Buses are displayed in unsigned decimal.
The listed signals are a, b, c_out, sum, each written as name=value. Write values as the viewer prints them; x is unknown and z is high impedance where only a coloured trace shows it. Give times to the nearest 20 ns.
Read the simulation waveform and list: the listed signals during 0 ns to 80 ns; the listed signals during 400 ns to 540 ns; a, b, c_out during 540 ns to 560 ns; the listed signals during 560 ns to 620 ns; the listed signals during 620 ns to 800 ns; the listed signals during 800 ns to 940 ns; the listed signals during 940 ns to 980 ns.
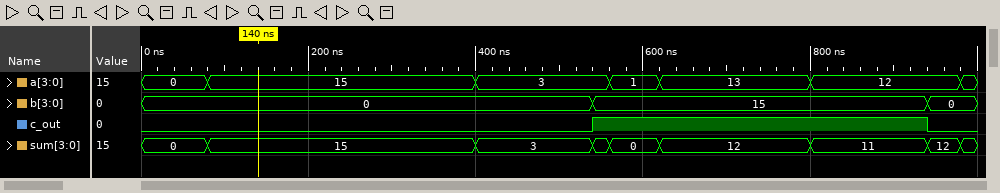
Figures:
a=0, b=0, c_out=0, sum=0
a=3, b=0, c_out=0, sum=3
a=3, b=15, c_out=1
a=1, b=15, c_out=1, sum=0
a=13, b=15, c_out=1, sum=12
a=12, b=15, c_out=1, sum=11
a=12, b=0, c_out=0, sum=12
